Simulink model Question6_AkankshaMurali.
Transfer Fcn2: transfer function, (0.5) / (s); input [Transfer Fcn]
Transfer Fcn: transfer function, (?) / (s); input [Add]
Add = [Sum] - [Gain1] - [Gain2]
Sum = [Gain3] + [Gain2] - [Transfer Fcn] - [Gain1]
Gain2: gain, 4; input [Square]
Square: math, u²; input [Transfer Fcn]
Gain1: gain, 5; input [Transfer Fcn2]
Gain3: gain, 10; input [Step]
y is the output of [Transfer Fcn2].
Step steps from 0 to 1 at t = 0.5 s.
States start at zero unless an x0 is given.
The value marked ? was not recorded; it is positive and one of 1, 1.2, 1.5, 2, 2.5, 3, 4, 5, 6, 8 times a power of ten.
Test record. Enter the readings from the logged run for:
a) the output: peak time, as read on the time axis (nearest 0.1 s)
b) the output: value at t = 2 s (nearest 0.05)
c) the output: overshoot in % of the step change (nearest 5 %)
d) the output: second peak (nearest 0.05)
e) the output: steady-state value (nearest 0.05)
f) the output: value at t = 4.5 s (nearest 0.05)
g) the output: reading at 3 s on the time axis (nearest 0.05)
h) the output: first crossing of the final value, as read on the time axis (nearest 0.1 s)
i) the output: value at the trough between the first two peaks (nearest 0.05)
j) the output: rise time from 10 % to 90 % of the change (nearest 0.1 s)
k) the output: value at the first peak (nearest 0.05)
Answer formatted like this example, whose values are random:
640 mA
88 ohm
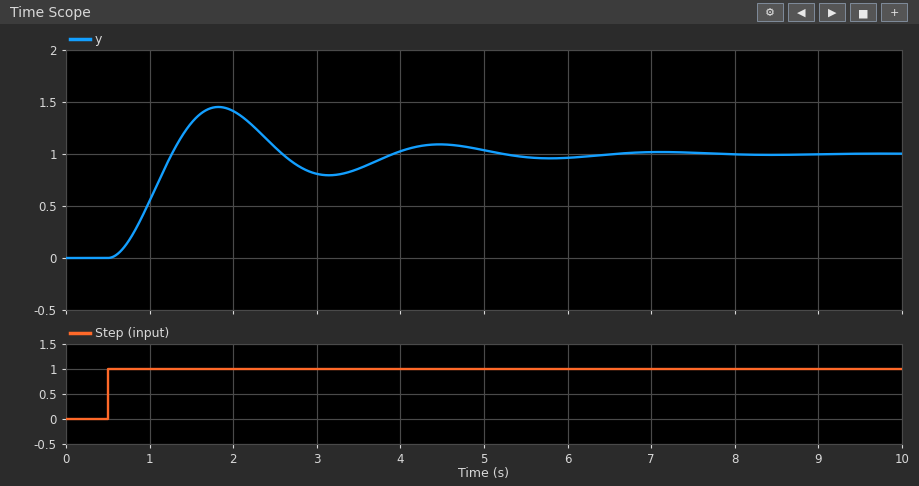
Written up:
1.8 s
1.40
45 %
1.10
1.00
1.10
0.80
1.3 s
0.80
0.5 s
1.45
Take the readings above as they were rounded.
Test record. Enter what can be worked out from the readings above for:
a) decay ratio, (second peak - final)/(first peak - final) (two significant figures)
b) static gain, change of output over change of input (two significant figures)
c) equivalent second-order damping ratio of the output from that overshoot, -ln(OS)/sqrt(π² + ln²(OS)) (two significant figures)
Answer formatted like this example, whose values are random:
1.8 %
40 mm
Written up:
0.22
1.0
0.25
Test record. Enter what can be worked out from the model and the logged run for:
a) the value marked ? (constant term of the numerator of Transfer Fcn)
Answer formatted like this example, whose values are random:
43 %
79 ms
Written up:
1.2
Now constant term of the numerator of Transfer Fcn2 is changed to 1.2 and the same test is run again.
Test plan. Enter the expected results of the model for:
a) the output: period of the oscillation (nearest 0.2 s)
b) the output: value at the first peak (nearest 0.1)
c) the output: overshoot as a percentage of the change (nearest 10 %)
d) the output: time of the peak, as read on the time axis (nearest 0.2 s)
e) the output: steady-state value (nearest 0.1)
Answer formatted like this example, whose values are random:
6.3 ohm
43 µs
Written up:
1.6 s
1.6
60 %
1.4 s
1.0
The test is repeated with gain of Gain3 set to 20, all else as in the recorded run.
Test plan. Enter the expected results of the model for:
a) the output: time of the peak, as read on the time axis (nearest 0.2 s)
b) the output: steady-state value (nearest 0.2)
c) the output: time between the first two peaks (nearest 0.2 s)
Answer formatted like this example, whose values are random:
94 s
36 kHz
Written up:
1.8 s
2.0
2.6 s
